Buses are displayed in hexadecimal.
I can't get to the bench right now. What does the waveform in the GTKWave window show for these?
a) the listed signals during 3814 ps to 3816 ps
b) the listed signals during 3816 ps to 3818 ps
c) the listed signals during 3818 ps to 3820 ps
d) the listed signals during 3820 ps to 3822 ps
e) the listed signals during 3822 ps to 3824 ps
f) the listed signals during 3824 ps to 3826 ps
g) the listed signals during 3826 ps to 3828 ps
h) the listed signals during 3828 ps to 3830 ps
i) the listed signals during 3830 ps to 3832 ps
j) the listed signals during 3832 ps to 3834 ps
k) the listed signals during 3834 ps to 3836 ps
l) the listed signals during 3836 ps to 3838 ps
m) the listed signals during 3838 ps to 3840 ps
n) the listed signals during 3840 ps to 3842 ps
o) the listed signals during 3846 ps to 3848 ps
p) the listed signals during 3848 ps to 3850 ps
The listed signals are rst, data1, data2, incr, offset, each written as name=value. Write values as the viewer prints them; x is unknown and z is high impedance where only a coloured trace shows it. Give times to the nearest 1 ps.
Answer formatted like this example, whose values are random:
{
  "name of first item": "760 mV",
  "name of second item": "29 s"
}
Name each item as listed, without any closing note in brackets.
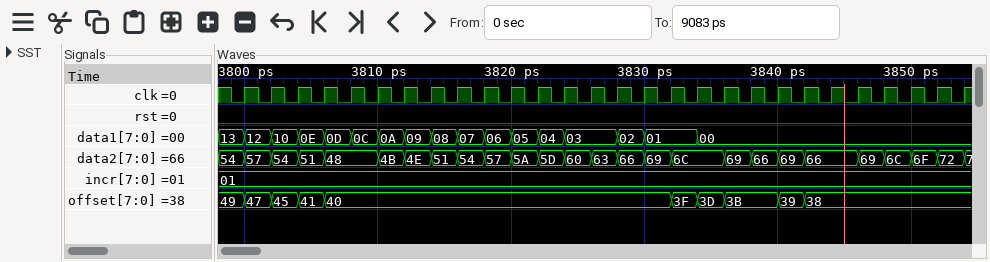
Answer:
{
  "the listed signals during 3814 ps to 3816 ps": "rst=0, data1=08, data2=51, incr=01, offset=40",
  "the listed signals during 3816 ps to 3818 ps": "rst=0, data1=07, data2=54, incr=01, offset=40",
  "the listed signals during 3818 ps to 3820 ps": "rst=0, data1=06, data2=57, incr=01, offset=40",
  "the listed signals during 3820 ps to 3822 ps": "rst=0, data1=05, data2=5A, incr=01, offset=40",
  "the listed signals during 3822 ps to 3824 ps": "rst=0, data1=04, data2=5D, incr=01, offset=40",
  "the listed signals during 3824 ps to 3826 ps": "rst=0, data1=03, data2=60, incr=01, offset=40",
  "the listed signals during 3826 ps to 3828 ps": "rst=0, data1=03, data2=63, incr=01, offset=40",
  "the listed signals during 3828 ps to 3830 ps": "rst=0, data1=02, data2=66, incr=01, offset=40",
  "the listed signals during 3830 ps to 3832 ps": "rst=0, data1=01, data2=69, incr=01, offset=40",
  "the listed signals during 3832 ps to 3834 ps": "rst=0, data1=01, data2=6C, incr=01, offset=3F",
  "the listed signals during 3834 ps to 3836 ps": "rst=0, data1=00, data2=6C, incr=01, offset=3D",
  "the listed signals during 3836 ps to 3838 ps": "rst=0, data1=00, data2=69, incr=01, offset=3B",
  "the listed signals during 3838 ps to 3840 ps": "rst=0, data1=00, data2=66, incr=01, offset=3B",
  "the listed signals during 3840 ps to 3842 ps": "rst=0, data1=00, data2=69, incr=01, offset=39",
  "the listed signals during 3846 ps to 3848 ps": "rst=0, data1=00, data2=69, incr=01, offset=38",
  "the listed signals during 3848 ps to 3850 ps": "rst=0, data1=00, data2=6C, incr=01, offset=38"
}
